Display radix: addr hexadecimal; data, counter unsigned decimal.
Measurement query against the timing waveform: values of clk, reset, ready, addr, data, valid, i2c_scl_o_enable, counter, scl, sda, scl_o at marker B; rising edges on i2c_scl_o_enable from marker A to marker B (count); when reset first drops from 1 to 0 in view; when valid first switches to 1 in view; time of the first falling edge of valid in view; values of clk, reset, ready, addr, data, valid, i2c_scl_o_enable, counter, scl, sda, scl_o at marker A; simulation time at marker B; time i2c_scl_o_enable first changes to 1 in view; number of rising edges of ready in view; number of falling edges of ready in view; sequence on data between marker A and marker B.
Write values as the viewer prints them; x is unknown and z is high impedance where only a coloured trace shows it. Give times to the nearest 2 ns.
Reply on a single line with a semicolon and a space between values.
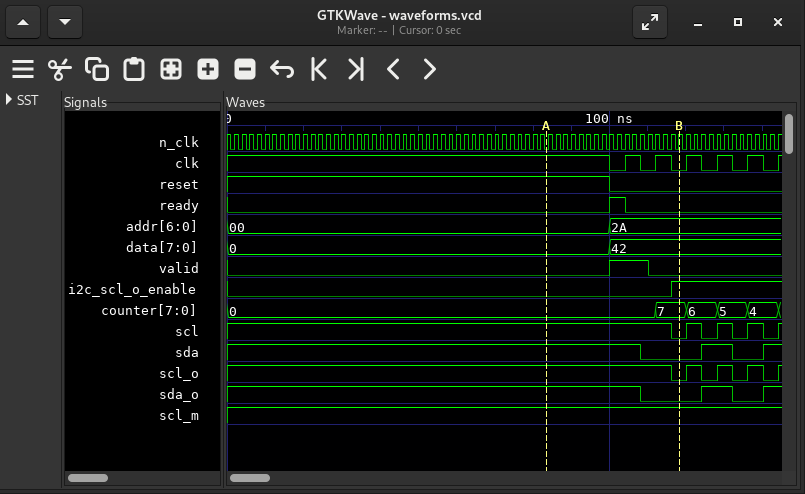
clk=0, reset=0, ready=0, addr=2A, data=42, valid=0, i2c_scl_o_enable=1, counter=7, scl=0, sda=0, scl_o=0; 1; 100 ns; 100 ns; 110 ns; clk=1, reset=1, ready=0, addr=00, data=0, valid=0, i2c_scl_o_enable=0, counter=0, scl=1, sda=1, scl_o=1; 118 ns; 116 ns; 1; 1; 0, 42
